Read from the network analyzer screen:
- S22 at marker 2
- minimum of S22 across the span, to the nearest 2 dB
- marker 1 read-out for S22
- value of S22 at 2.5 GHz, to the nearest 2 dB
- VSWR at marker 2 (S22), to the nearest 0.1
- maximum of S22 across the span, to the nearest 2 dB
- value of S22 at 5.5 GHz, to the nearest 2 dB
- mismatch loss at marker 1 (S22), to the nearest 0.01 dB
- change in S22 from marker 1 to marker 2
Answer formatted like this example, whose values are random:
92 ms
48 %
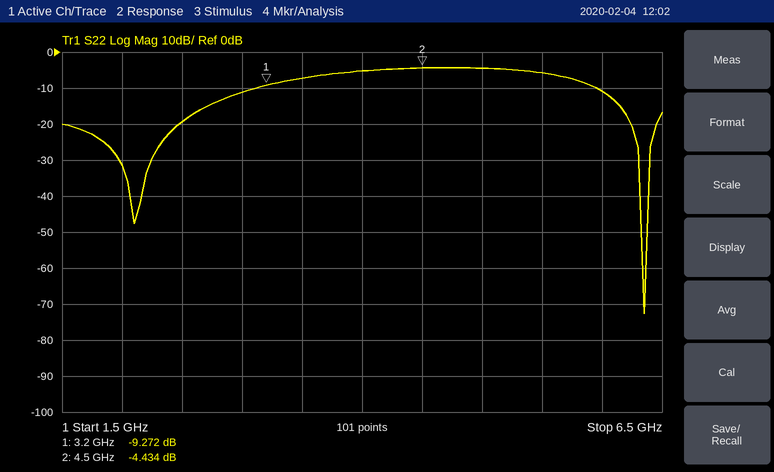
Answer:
-4.434 dB
-72 dB
-9.272 dB
-20 dB
4.0
-4 dB
-6 dB
0.55 dB
4.838 dB
